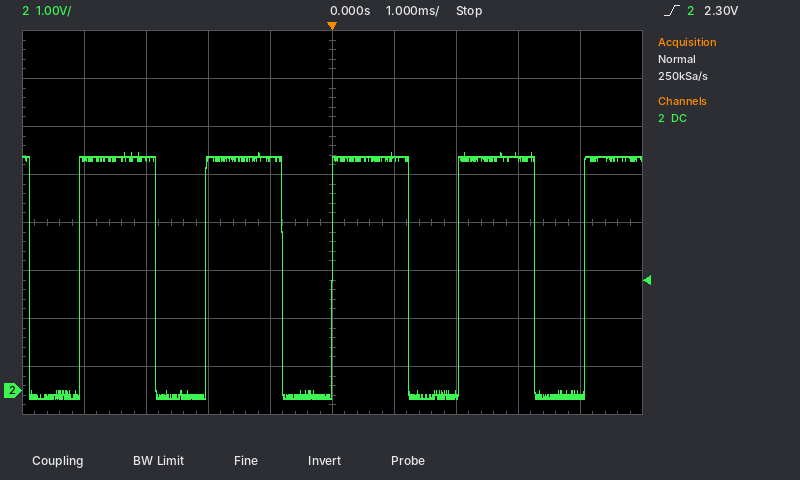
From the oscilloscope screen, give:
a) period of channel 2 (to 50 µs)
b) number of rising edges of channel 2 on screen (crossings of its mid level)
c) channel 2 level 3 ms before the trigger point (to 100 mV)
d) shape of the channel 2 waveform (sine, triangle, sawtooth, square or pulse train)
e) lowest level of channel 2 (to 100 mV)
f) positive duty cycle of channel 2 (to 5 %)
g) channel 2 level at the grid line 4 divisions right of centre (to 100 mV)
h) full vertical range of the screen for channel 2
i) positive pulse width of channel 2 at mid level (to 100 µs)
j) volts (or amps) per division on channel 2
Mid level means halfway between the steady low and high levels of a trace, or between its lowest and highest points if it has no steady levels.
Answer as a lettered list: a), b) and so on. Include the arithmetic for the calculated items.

a) 2.05 ms
b) 5
c) 4.8 V
d) pulse train
e) -200 mV
f) 1.2 ms / 2.05 ms ≈ 58.5 %, so 60 % to the nearest 5 %
g) -100 mV
h) 8 V
i) 1.2 ms
j) 1 V
